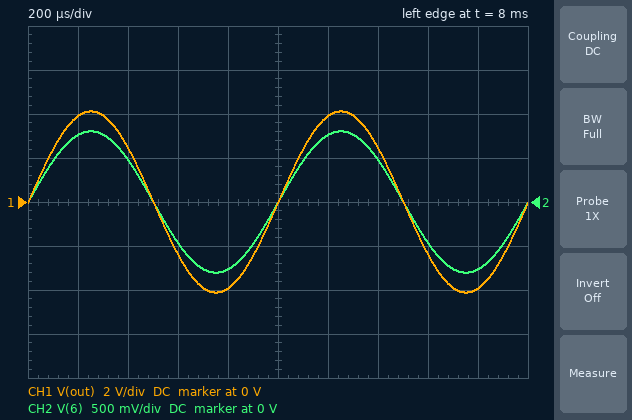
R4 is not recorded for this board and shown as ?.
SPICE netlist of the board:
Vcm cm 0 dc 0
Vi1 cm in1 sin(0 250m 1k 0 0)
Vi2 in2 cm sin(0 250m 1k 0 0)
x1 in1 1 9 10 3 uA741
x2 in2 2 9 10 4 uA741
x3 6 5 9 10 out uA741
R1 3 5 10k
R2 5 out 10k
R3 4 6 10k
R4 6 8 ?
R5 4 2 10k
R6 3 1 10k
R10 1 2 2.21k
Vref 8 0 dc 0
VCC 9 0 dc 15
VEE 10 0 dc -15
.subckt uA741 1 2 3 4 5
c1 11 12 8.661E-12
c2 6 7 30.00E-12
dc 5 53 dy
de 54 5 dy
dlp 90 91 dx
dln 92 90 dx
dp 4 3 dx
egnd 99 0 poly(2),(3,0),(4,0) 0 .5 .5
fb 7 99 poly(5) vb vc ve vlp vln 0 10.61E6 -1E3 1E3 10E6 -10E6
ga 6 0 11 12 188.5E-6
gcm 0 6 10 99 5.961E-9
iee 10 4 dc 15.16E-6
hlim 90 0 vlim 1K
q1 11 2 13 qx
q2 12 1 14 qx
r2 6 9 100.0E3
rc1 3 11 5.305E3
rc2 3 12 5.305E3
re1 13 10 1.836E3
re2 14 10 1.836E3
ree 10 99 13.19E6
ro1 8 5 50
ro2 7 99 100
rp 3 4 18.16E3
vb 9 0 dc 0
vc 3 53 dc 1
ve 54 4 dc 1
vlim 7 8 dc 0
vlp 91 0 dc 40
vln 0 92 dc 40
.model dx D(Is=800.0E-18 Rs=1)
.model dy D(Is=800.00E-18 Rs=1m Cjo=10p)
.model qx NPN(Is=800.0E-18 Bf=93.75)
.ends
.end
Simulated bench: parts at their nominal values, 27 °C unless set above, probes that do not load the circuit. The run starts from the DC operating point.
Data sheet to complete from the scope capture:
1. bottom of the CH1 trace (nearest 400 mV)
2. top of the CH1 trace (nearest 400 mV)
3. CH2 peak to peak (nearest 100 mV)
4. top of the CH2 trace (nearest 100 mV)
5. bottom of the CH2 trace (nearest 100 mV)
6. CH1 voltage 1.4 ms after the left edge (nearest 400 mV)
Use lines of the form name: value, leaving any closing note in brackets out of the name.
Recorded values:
bottom of the CH1 trace: -4.0 V
top of the CH1 trace: 4.0 V
CH2 peak to peak: 1.6 V
top of the CH2 trace: 800 mV
bottom of the CH2 trace: -800 mV
CH1 voltage 1.4 ms after the left edge: 2.4 V
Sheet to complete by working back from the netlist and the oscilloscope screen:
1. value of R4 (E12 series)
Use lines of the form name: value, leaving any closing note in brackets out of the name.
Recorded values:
value of R4: 4.7 kΩ
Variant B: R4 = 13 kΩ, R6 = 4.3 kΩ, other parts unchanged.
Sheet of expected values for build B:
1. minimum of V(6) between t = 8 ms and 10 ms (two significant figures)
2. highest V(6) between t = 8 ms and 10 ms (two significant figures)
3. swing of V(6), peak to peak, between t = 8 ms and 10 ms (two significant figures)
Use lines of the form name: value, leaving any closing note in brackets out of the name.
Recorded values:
minimum of V(6) between t = 8 ms and 10 ms: -1.4 V
highest V(6) between t = 8 ms and 10 ms: 1.4 V
swing of V(6), peak to peak, between t = 8 ms and 10 ms: 2.8 V
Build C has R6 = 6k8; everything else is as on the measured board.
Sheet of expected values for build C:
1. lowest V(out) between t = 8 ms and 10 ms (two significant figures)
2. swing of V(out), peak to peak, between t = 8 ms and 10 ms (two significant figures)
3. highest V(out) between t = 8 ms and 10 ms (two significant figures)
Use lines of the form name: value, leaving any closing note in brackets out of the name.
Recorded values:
lowest V(out) between t = 8 ms and 10 ms: -3.4 V
swing of V(out), peak to peak, between t = 8 ms and 10 ms: 6.8 V
highest V(out) between t = 8 ms and 10 ms: 3.4 V
